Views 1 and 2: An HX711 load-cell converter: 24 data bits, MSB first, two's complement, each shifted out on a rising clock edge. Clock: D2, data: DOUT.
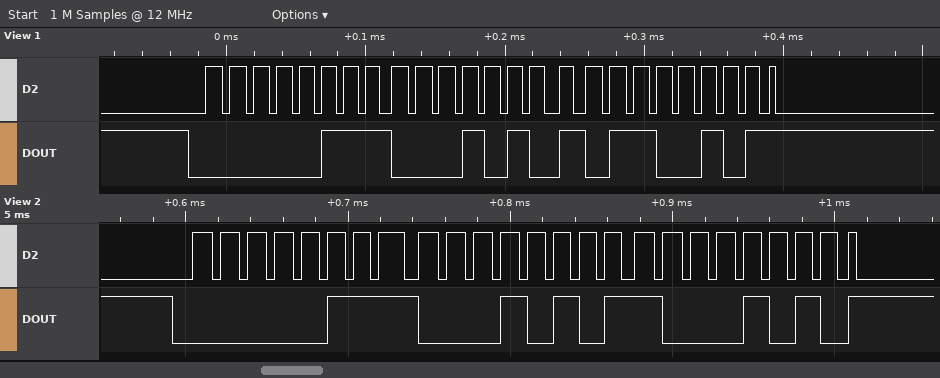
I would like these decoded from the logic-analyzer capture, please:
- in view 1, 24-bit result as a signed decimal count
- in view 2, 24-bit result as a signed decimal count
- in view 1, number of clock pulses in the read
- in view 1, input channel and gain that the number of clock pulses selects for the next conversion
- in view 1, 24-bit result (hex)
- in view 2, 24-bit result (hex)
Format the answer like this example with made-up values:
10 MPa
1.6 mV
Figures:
464229
464266
25
channel A, gain 128
0x071565
0x07158A
